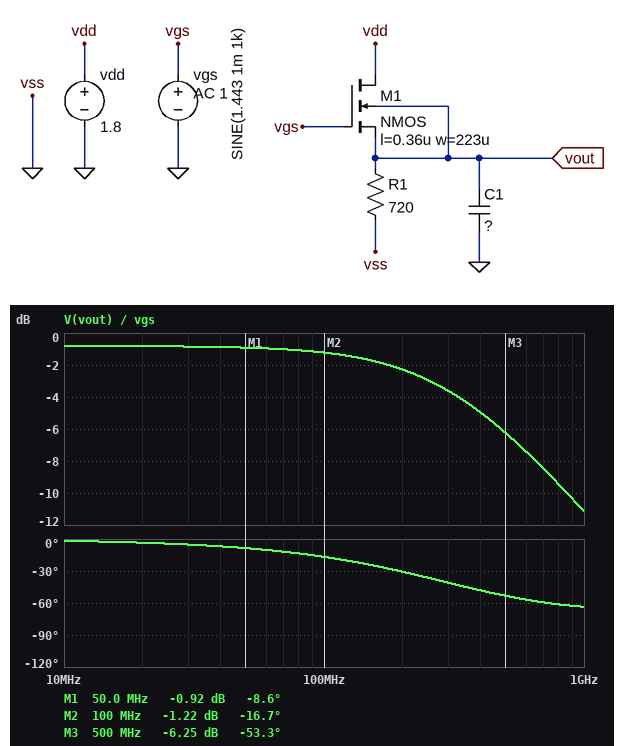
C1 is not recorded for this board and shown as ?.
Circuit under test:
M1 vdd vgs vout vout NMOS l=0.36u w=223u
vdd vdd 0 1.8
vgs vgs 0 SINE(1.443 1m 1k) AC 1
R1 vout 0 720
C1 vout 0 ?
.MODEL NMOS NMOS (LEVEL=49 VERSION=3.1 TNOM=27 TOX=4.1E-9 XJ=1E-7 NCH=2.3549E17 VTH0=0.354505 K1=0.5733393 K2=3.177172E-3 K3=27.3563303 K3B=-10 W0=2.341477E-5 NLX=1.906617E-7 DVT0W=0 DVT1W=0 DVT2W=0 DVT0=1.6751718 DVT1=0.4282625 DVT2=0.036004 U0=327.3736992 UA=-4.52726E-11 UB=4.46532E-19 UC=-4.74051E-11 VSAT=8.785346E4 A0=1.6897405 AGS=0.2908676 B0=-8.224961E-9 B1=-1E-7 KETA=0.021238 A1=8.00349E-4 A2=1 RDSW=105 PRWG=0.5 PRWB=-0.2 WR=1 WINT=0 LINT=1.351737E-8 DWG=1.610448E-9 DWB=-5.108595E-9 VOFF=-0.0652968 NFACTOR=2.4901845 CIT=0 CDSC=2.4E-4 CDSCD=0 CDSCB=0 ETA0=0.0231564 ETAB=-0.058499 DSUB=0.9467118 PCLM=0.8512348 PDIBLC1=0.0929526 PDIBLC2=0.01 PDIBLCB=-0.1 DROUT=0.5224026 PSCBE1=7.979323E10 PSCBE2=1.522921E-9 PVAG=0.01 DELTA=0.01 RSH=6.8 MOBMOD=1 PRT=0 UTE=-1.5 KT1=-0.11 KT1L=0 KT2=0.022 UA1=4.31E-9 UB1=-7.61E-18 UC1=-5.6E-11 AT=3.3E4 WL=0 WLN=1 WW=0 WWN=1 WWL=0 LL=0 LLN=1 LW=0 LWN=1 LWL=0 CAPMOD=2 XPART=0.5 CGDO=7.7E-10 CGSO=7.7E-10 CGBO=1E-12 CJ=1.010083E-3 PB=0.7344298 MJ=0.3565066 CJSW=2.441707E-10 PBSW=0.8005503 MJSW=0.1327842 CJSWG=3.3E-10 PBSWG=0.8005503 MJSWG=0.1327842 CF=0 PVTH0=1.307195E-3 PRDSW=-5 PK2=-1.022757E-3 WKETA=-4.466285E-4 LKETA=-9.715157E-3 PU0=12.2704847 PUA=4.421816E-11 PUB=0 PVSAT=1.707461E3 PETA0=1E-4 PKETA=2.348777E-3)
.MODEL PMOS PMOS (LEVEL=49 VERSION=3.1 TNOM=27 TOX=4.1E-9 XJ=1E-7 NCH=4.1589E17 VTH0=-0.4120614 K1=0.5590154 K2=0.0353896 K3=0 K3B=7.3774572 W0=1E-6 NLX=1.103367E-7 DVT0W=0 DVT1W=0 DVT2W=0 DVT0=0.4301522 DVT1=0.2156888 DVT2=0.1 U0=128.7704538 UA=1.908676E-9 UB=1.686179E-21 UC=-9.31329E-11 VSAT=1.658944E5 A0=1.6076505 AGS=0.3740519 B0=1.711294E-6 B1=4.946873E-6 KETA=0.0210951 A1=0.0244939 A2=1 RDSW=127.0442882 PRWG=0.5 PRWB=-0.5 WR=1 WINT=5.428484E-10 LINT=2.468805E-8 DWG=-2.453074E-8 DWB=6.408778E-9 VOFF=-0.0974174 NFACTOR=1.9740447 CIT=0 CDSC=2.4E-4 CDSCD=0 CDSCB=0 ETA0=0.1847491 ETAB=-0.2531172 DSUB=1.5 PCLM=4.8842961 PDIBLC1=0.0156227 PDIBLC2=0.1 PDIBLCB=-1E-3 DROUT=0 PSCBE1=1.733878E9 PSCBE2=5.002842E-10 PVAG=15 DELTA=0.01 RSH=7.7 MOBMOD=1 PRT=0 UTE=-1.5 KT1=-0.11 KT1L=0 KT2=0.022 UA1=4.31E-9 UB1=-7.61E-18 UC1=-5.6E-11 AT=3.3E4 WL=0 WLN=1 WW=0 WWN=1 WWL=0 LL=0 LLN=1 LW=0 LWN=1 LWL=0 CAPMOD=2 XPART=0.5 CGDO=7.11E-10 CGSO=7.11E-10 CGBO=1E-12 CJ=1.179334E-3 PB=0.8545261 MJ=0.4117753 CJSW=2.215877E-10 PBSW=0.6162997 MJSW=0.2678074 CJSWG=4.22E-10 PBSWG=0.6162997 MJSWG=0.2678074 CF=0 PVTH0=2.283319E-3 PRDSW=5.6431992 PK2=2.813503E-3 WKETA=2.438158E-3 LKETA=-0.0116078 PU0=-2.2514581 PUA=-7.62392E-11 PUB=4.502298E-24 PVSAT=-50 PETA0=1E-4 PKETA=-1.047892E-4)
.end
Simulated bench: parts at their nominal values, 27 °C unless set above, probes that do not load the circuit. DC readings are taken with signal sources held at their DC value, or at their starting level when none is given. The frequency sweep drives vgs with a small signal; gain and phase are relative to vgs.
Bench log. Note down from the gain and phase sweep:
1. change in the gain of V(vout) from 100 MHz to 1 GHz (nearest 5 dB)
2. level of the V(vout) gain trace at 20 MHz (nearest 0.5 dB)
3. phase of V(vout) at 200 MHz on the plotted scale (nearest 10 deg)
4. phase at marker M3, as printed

-10 dB
-1.0 dB
-30 deg
-53.3 deg
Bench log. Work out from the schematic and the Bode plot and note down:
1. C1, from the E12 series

8.2 pF
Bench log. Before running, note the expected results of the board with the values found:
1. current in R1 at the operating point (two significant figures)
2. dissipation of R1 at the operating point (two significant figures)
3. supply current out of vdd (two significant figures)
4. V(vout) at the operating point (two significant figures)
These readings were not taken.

1.2 mA
960 µW
1.2 mA
830 mV
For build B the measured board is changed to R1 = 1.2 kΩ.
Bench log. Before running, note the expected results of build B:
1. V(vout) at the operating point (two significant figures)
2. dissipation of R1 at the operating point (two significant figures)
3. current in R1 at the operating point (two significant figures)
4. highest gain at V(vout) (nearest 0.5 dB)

860 mV
620 µW
720 µA
-0.5 dB
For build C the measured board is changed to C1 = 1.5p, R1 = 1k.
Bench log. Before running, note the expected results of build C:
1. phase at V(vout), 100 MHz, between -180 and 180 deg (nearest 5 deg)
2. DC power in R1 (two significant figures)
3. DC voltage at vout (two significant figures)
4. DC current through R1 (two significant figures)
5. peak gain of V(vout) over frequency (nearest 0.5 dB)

-5 deg
730 µW
850 mV
850 µA
-0.5 dB
